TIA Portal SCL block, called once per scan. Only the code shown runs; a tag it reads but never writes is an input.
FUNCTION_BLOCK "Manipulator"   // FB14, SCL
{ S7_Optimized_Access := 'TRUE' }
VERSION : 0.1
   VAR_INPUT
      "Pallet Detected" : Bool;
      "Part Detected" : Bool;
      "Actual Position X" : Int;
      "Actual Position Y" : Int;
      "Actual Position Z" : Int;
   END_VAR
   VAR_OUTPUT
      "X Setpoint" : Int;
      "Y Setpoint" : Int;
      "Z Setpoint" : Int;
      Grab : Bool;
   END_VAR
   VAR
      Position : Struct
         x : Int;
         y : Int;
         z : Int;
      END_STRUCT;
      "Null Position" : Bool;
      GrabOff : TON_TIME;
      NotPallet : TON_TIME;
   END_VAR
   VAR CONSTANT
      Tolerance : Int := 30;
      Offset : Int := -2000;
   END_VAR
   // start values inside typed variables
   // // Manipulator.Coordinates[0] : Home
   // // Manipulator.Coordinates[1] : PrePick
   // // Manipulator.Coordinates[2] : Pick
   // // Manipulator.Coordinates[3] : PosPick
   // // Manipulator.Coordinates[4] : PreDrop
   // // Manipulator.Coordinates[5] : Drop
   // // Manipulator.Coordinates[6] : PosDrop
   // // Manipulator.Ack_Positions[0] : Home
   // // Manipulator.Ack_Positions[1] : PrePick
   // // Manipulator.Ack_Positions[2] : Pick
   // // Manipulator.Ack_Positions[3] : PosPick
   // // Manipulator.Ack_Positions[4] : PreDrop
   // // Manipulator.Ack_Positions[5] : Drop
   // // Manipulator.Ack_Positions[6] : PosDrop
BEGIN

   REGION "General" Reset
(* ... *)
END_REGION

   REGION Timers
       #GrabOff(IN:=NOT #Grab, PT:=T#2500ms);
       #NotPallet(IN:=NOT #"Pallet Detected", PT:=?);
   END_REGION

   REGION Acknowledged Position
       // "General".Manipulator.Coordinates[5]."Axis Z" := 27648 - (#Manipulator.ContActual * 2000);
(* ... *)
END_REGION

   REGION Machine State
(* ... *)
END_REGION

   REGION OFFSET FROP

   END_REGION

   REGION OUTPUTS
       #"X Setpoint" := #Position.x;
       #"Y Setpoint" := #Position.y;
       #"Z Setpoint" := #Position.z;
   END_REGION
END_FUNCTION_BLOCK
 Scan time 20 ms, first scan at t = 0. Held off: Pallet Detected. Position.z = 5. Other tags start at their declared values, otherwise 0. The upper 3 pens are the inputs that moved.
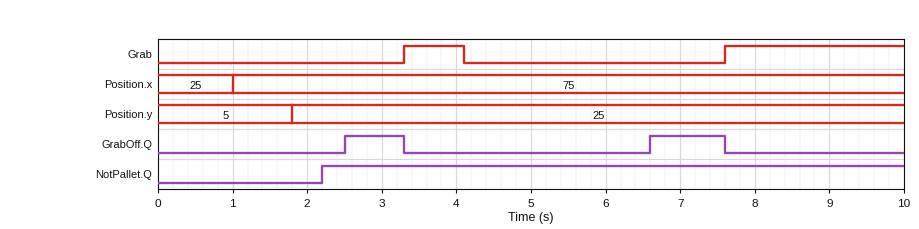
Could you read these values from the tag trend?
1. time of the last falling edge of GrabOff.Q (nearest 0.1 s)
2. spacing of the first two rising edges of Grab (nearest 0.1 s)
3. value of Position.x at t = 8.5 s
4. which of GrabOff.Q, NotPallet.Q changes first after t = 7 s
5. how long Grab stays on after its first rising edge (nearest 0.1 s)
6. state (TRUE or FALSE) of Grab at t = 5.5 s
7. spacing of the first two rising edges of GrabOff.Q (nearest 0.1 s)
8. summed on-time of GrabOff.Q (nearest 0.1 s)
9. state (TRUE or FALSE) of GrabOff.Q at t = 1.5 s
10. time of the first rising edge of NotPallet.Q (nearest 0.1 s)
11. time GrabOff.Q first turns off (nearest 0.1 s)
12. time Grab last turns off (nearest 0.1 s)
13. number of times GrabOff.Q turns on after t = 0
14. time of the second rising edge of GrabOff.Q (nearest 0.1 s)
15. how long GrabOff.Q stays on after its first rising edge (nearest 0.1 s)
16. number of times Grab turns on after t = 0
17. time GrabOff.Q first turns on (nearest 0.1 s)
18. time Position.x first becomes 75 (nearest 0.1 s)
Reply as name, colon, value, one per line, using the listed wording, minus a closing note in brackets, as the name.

time of the last falling edge of GrabOff.Q: 7.6 s
spacing of the first two rising edges of Grab: 4.3 s
value of Position.x at t = 8.5 s: 75
which of GrabOff.Q, NotPallet.Q changes first after t = 7 s: GrabOff.Q
how long Grab stays on after its first rising edge: 0.8 s
state (TRUE or FALSE) of Grab at t = 5.5 s: FALSE
spacing of the first two rising edges of GrabOff.Q: 4.1 s
summed on-time of GrabOff.Q: 1.8 s
state (TRUE or FALSE) of GrabOff.Q at t = 1.5 s: FALSE
time of the first rising edge of NotPallet.Q: 2.2 s
time GrabOff.Q first turns off: 3.3 s
time Grab last turns off: 4.1 s
number of times GrabOff.Q turns on after t = 0: 2
time of the second rising edge of GrabOff.Q: 6.6 s
how long GrabOff.Q stays on after its first rising edge: 0.8 s
number of times Grab turns on after t = 0: 2
time GrabOff.Q first turns on: 2.5 s
time Position.x first becomes 75: 1.0 s
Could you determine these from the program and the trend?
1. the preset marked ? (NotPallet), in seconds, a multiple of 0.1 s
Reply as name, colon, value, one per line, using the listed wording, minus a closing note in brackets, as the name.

the preset marked ? (NotPallet), in seconds, a multiple of 0.1 s: 2.2 s
